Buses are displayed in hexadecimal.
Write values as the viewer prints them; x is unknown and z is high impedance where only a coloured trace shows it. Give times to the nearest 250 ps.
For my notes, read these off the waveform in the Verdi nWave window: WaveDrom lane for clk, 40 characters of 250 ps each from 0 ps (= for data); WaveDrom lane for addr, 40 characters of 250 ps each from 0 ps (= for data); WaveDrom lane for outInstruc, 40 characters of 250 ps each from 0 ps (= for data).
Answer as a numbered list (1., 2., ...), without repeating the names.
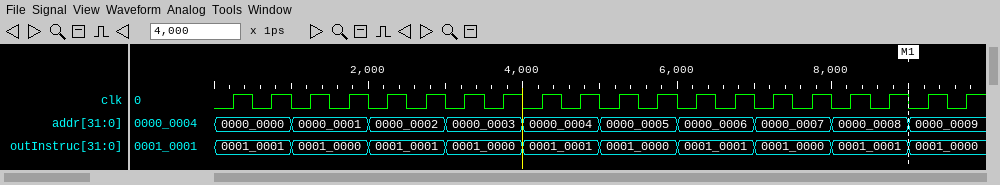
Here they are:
1. {name: 'clk', wave: '0101010101010101010101010101010101010101'}
2. {name: 'addr', wave: '=...=...=...=...=...=...=...=...=...=...', data: '0000_0000 0000_0001 0000_0002 0000_0003 0000_0004 0000_0005 0000_0006 0000_0007 0000_0008 0000_0009'}
3. {name: 'outInstruc', wave: '=...=...=...=...=...=...=...=...=...=...', data: '0001_0001 0001_0000 0001_0001 0001_0000 0001_0001 0001_0000 0001_0001 0001_0000 0001_0001 0001_0000'}
